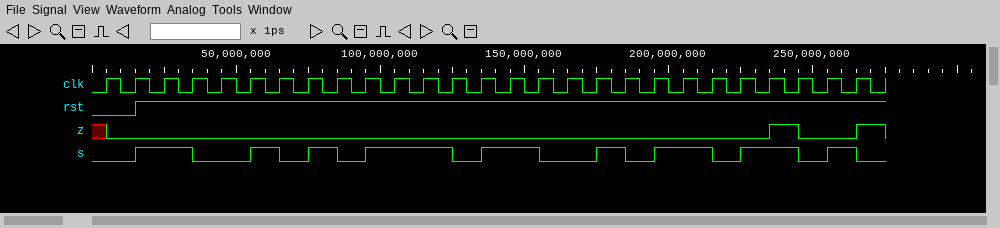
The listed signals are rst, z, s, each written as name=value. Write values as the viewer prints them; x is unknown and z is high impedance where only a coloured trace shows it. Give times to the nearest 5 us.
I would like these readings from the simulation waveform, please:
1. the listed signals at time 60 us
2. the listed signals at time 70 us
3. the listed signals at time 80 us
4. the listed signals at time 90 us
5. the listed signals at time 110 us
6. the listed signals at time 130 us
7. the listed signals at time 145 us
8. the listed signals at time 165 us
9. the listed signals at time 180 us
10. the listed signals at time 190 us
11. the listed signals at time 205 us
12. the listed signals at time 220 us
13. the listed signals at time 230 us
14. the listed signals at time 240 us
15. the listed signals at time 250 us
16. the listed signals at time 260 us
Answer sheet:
rst=1, z=0, s=1
rst=1, z=0, s=0
rst=1, z=0, s=1
rst=1, z=0, s=0
rst=1, z=0, s=1
rst=1, z=0, s=0
rst=1, z=0, s=1
rst=1, z=0, s=0
rst=1, z=0, s=1
rst=1, z=0, s=0
rst=1, z=0, s=1
rst=1, z=0, s=0
rst=1, z=0, s=1
rst=1, z=1, s=1
rst=1, z=0, s=0
rst=1, z=0, s=1
